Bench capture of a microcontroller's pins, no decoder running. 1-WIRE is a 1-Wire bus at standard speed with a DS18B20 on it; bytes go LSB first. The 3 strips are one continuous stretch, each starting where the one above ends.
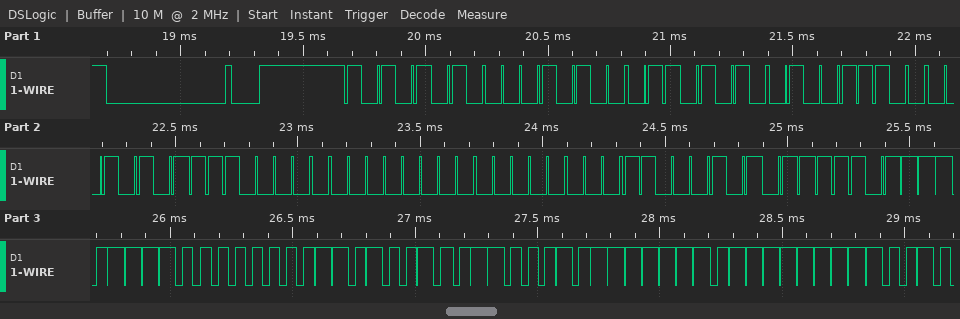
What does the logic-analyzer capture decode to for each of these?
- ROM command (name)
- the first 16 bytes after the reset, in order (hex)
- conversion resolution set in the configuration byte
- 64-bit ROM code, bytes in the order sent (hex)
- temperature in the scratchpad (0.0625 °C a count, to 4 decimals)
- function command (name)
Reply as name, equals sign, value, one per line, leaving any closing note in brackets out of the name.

ROM command = Match ROM
the first 16 bytes after the reset, in order = 55 28 56 72 A8 07 00 00 A3 BE F7 00 4B 46 7F FF
conversion resolution set in the configuration byte = 12 bits
64-bit ROM code, bytes in the order sent = 28 56 72 A8 07 00 00 A3
temperature in the scratchpad = 15.4375 °C
function command = Read Scratchpad
